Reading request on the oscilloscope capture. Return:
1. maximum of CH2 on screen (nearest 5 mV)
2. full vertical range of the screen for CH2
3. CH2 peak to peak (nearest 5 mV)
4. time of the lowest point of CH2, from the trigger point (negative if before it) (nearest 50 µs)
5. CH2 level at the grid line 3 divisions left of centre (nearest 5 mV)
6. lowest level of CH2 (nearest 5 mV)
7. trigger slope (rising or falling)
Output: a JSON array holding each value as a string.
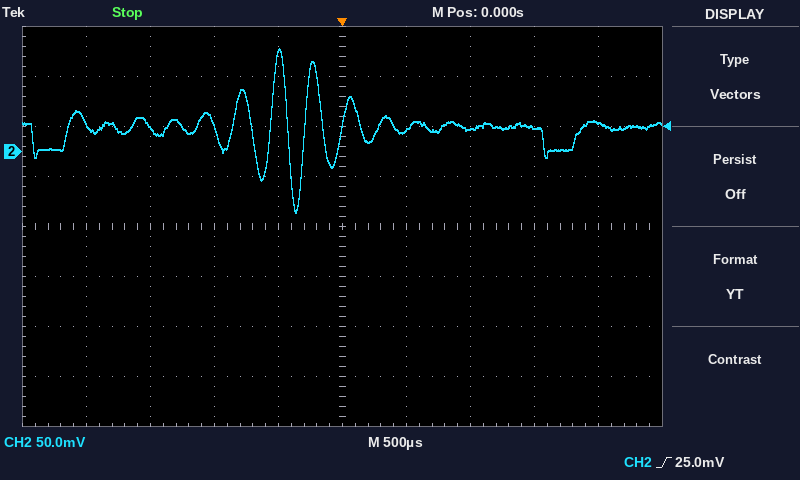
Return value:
["105 mV", "400 mV", "165 mV", "-350 µs", "25 mV", "-60 mV", "rising"]
